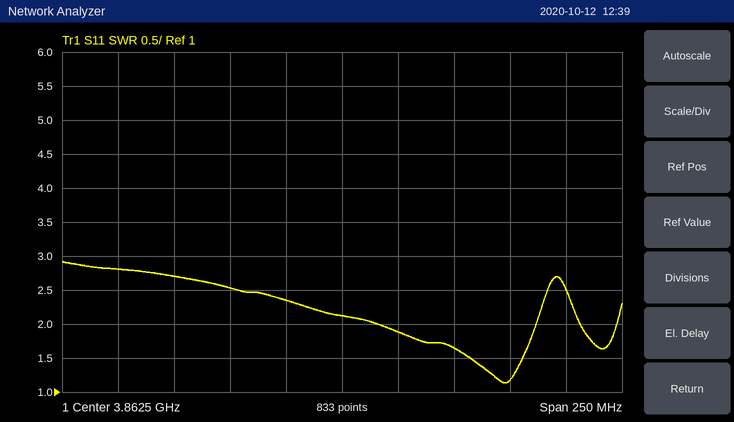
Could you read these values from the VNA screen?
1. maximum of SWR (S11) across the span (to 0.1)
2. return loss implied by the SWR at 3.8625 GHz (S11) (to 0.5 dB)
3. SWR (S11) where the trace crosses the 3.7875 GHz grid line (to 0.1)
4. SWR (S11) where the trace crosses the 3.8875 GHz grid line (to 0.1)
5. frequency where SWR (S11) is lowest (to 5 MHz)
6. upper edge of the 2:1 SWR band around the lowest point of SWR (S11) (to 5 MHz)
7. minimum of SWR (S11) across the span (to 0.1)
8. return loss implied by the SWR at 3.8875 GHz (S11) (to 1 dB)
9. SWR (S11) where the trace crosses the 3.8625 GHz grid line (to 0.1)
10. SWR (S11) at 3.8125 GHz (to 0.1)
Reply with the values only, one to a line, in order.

2.9
9.0 dB
2.7
1.9
3.935 GHz
3.950 GHz
1.1
10 dB
2.1
2.5
